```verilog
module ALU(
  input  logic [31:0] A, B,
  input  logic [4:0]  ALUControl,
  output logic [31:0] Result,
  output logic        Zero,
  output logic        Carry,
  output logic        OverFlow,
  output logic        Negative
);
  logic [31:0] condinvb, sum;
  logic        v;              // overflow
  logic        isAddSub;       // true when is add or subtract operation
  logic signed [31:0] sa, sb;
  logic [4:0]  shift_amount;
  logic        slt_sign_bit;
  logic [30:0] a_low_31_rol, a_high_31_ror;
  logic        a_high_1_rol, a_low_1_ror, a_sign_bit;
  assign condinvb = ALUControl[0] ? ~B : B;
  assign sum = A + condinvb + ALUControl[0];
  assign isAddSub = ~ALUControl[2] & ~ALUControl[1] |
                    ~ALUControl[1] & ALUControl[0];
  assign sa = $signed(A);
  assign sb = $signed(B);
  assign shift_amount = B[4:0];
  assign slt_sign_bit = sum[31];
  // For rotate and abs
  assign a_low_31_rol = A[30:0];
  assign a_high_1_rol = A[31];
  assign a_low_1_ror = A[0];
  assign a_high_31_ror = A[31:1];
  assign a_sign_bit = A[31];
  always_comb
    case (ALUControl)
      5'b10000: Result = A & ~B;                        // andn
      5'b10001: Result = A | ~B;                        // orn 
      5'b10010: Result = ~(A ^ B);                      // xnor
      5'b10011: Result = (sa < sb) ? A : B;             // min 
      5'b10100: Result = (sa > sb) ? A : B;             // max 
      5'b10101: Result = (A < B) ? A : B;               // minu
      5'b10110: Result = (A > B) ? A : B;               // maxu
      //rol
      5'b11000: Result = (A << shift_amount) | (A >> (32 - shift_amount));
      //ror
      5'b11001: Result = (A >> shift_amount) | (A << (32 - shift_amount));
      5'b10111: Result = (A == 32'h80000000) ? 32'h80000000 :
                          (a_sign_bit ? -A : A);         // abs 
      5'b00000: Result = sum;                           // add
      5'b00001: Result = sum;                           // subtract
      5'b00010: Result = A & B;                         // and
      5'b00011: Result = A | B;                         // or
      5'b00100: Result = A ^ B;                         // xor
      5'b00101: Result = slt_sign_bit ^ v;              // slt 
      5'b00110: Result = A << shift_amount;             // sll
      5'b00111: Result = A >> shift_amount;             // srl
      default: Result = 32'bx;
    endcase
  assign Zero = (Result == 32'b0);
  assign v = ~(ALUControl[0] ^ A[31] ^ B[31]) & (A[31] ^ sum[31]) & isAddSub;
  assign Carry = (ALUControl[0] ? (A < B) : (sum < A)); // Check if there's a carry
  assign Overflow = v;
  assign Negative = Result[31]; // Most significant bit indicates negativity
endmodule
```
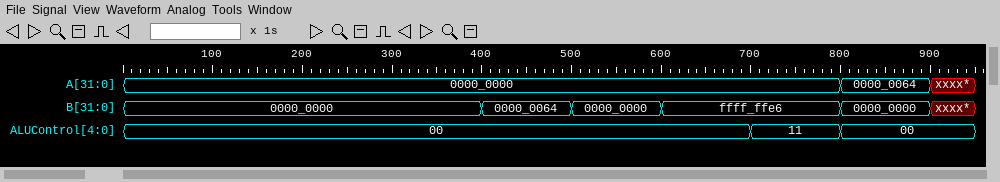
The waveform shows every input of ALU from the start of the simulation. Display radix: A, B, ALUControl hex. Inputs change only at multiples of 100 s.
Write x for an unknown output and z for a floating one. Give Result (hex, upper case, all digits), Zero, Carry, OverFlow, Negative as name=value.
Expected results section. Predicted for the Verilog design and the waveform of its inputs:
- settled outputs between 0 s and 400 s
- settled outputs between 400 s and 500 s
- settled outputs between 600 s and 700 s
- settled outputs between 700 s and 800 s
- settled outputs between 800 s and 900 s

Result=00000000, Zero=1, Carry=0, OverFlow=x, Negative=0
Result=00000064, Zero=0, Carry=0, OverFlow=x, Negative=0
Result=FFFFFFE6, Zero=0, Carry=0, OverFlow=x, Negative=1
Result=00000019, Zero=0, Carry=1, OverFlow=x, Negative=0
Result=00000064, Zero=0, Carry=0, OverFlow=x, Negative=0
